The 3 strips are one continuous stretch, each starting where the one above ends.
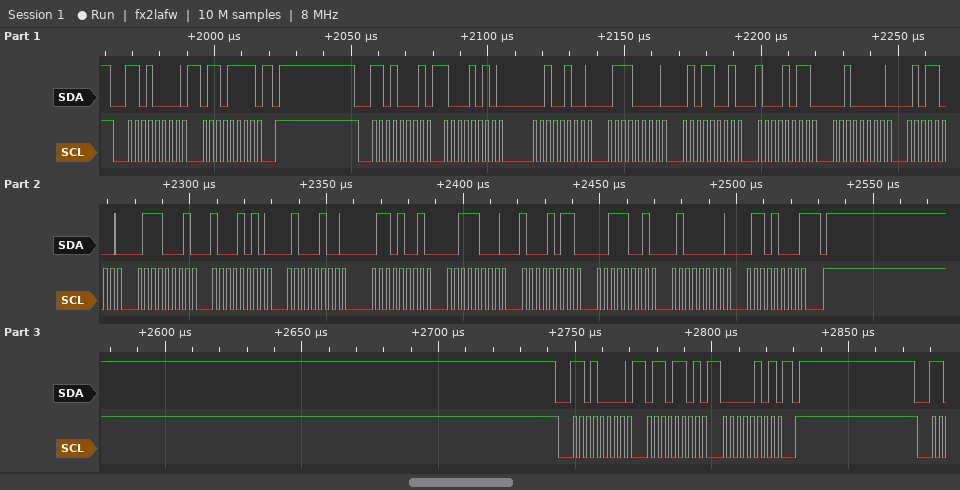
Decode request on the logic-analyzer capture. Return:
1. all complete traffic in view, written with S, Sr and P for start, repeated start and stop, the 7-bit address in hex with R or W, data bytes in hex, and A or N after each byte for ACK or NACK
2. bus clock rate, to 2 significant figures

S 68W A 6F A P S 68R A 8A A 24 A 70 A 59 A 8B A 20 A 58 A 71 A 8A A 44 A 69 A 38 A 8B A 39 A 40 A 68 N P S 68W A 6D A 05 A P
400 kHz
